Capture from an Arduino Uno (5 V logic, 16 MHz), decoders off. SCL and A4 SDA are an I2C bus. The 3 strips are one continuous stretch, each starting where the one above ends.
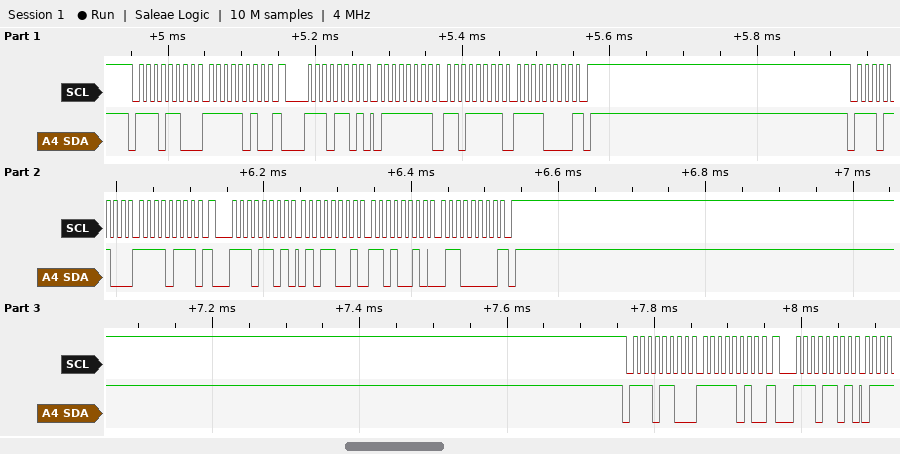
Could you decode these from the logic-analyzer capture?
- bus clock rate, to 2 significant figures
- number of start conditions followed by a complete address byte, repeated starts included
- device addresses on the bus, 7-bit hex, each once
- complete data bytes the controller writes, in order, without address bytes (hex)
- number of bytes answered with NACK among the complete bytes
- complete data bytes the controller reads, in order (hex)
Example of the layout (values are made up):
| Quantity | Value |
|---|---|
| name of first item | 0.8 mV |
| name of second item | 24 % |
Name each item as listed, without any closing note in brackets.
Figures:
| Quantity | Value |
|---|---|
| bus clock rate, to 2 significant figures | 100 kHz |
| number of start conditions followed by a complete address byte, repeated starts included | 6 |
| device addresses on the bus, 7-bit hex, each once | 0x76 |
| complete data bytes the controller writes, in order, without address bytes | FA F7 FA |
| number of bytes answered with NACK among the complete bytes | 2 |
| complete data bytes the controller reads, in order | 7F DF F0 59 D2 60 |
